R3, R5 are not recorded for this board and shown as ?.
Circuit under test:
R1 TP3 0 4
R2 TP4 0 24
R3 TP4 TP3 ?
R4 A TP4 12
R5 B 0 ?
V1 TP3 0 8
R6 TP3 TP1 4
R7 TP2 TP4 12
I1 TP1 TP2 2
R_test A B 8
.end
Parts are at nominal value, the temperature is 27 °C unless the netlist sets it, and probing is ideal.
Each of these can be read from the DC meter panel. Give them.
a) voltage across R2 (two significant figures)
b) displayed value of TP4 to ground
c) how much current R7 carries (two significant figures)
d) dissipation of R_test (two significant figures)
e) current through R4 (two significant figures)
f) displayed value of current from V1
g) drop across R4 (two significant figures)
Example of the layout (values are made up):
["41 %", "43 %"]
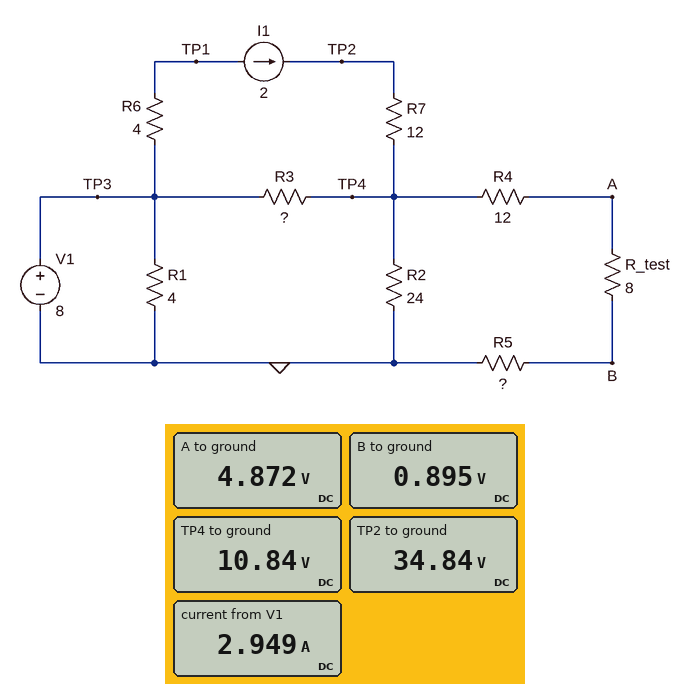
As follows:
["11 V", "10.84 V", "2.0 A", "2.0 W", "500 mA", "2.949 A", "6.0 V"]
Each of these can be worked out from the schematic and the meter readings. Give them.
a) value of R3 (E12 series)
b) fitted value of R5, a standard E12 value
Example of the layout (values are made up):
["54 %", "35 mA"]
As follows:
["2.7 Ω", "1.8 Ω"]
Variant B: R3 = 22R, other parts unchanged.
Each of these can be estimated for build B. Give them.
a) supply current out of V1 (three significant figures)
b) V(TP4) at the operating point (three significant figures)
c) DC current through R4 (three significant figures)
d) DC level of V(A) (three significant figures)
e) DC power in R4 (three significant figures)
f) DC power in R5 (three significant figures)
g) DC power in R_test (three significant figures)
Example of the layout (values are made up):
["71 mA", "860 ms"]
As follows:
["3.56 A", "17.8 V", "815 mA", "7.99 V", "7.98 W", "1.20 W", "5.32 W"]
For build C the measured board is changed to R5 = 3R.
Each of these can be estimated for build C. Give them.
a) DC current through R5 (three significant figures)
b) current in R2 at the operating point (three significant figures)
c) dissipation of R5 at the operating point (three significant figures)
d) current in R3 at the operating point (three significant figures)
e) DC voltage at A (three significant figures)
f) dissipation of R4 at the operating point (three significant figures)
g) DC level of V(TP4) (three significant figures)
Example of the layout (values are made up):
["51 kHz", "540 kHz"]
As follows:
["474 mA", "454 mA", "673 mW", "1.07 A", "5.21 V", "2.69 W", "10.9 V"]
